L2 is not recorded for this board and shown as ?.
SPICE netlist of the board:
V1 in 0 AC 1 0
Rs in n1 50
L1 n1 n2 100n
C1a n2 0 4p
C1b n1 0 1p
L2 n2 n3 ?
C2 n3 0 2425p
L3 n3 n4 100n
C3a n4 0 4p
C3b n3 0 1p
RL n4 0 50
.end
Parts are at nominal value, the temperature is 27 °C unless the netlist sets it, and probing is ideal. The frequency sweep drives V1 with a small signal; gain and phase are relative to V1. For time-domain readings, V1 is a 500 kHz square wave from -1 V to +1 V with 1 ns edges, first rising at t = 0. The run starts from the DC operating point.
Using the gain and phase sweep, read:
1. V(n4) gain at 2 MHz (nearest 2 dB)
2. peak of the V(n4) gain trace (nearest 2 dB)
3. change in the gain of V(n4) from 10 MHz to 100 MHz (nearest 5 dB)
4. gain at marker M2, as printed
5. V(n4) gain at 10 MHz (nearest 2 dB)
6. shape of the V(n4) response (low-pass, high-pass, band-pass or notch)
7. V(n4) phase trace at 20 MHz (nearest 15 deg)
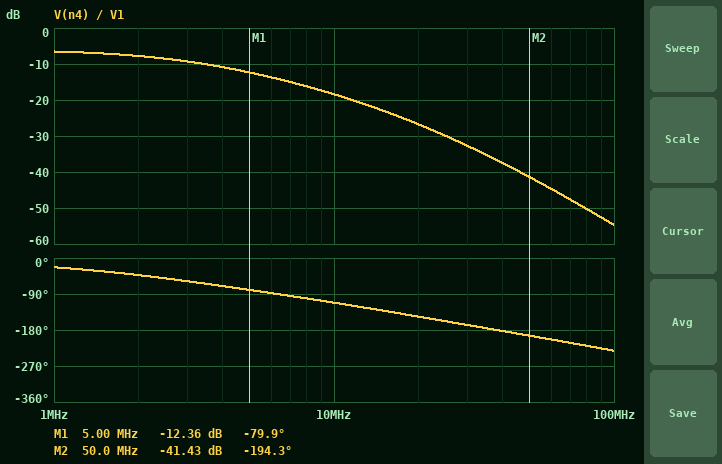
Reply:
-8 dB
-6 dB
-35 dB
-41.43 dB
-18 dB
low-pass
-150 deg
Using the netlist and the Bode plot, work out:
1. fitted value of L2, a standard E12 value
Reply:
330 nH
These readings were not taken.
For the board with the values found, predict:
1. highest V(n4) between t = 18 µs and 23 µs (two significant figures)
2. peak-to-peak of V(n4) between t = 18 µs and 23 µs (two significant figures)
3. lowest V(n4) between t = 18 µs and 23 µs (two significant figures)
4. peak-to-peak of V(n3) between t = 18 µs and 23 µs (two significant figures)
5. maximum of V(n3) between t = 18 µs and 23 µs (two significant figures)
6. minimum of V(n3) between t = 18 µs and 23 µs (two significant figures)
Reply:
500 mV
1.0 V
-500 mV
1.0 V
500 mV
-500 mV
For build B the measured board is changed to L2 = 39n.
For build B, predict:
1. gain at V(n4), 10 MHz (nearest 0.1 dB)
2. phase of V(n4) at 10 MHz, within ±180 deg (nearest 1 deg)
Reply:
-17.8 dB
-92 deg
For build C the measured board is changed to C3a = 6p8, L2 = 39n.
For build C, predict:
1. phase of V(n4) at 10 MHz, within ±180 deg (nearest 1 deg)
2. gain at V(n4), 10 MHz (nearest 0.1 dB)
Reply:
-92 deg
-17.8 dB
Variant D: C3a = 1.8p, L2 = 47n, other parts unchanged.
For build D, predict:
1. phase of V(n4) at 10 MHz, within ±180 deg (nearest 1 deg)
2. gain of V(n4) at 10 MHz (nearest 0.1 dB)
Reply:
-93 deg
-17.8 dB
